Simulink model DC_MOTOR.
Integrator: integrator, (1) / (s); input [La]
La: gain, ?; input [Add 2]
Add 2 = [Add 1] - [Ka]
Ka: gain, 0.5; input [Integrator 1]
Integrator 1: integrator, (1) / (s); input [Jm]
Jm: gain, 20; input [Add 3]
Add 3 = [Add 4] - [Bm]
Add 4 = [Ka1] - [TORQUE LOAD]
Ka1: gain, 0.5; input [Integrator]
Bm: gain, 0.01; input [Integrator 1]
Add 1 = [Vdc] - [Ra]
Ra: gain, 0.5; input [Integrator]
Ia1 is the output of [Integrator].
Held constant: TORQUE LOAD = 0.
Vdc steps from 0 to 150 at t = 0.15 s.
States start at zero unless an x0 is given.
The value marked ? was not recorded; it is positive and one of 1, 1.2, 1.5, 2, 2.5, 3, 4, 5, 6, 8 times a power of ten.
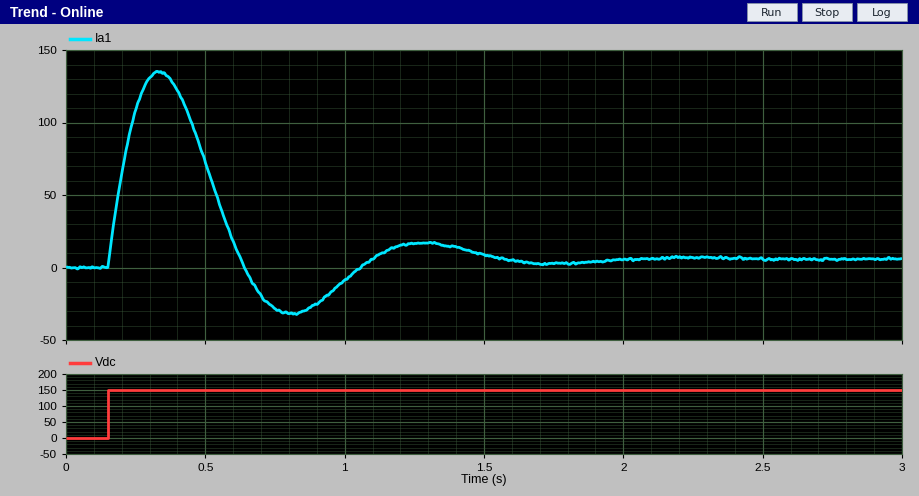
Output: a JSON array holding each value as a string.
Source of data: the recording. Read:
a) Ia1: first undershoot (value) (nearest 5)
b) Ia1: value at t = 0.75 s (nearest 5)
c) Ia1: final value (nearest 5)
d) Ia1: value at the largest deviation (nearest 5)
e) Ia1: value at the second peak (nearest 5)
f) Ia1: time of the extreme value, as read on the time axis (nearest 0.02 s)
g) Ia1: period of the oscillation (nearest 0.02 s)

["-30", "-30", "5", "135", "15", "0.34 s", "0.94 s"]
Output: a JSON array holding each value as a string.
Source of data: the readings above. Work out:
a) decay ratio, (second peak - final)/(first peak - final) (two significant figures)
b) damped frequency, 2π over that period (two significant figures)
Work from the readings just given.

["0.077", "6.7 rad/s"]
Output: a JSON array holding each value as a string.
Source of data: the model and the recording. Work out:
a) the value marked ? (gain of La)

["10"]
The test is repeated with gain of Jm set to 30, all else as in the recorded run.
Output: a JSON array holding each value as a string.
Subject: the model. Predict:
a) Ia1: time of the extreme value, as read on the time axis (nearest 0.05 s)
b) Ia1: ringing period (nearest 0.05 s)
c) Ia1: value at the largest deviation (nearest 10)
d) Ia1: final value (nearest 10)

["0.30 s", "0.75 s", "120", "10"]
